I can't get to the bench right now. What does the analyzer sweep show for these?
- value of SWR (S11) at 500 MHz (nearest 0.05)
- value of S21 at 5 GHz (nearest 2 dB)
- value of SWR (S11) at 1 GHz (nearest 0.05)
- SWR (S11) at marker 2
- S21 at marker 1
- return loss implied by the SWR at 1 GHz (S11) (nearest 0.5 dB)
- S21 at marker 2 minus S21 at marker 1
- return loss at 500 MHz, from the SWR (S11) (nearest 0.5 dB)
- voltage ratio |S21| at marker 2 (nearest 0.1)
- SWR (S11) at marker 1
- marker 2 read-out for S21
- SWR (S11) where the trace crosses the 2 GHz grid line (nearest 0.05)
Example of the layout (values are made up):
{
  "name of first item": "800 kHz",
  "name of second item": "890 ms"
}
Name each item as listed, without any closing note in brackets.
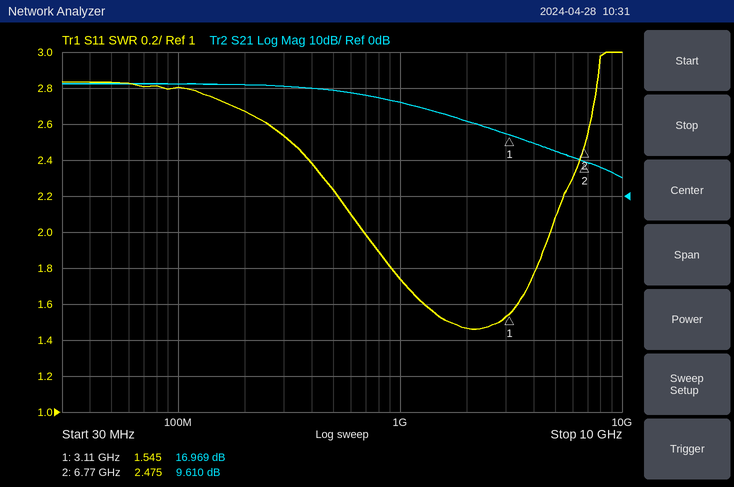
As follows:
{
  "value of SWR (S11) at 500 MHz": "2.25",
  "value of S21 at 5 GHz": "12 dB",
  "value of SWR (S11) at 1 GHz": "1.75",
  "SWR (S11) at marker 2": "2.475",
  "S21 at marker 1": "16.969 dB",
  "return loss implied by the SWR at 1 GHz (S11)": "11.5 dB",
  "S21 at marker 2 minus S21 at marker 1": "-7.359 dB",
  "return loss at 500 MHz, from the SWR (S11)": "8.5 dB",
  "voltage ratio |S21| at marker 2": "3.0",
  "SWR (S11) at marker 1": "1.545",
  "marker 2 read-out for S21": "9.610 dB",
  "SWR (S11) where the trace crosses the 2 GHz grid line": "1.45"
}
